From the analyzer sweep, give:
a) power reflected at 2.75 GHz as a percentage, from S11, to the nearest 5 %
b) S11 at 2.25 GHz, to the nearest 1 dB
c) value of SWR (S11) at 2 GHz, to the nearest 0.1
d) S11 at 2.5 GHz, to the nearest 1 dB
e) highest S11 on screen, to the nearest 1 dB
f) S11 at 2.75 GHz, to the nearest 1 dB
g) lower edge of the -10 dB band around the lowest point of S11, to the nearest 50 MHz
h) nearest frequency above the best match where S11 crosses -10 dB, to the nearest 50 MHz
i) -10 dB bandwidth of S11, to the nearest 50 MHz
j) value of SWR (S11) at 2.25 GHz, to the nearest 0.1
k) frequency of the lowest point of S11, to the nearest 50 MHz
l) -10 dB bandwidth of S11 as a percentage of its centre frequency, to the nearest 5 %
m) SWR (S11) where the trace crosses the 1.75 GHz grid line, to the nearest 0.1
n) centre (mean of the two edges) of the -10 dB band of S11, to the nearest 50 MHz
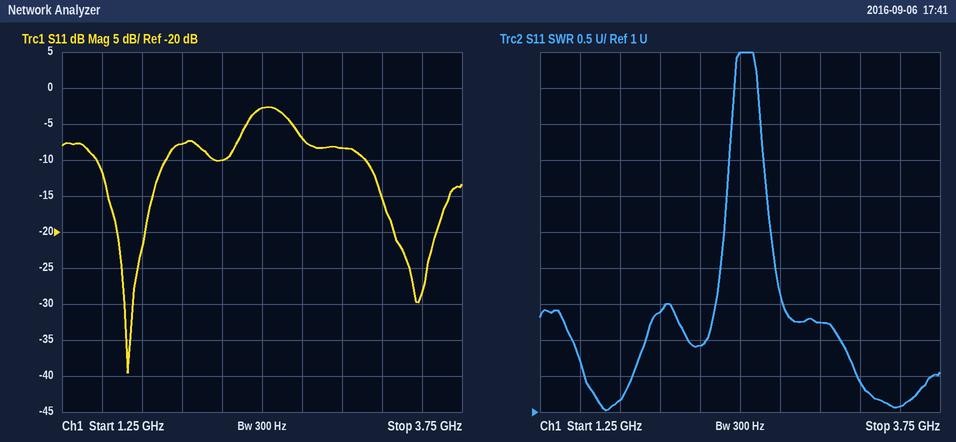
20 %
-10 dB
2.4
-3 dB
-3 dB
-7 dB
1.45 GHz
1.90 GHz
450 MHz
1.9
1.65 GHz
25 %
1.2
1.70 GHz
